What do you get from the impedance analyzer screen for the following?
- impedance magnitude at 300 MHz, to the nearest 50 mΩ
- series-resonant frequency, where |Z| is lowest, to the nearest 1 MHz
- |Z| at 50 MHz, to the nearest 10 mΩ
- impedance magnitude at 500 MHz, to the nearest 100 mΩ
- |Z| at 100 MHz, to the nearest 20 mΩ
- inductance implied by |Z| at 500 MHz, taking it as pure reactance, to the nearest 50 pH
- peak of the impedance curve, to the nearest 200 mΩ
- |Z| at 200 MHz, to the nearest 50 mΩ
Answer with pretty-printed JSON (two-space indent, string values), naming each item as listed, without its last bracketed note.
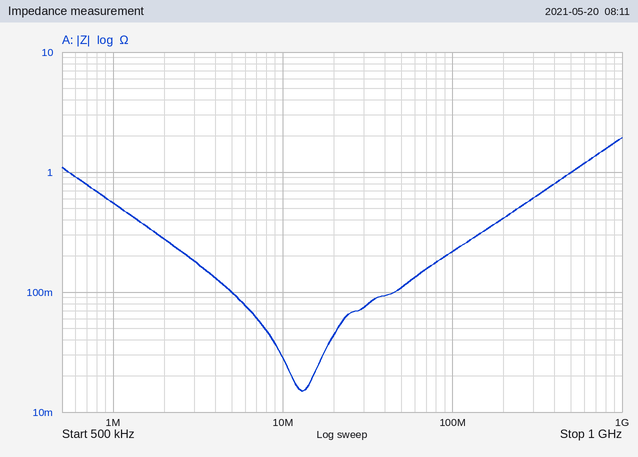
{
  "impedance magnitude at 300 MHz, to the nearest 50 mΩ": "600 mΩ",
  "series-resonant frequency, where |Z| is lowest, to the nearest 1 MHz": "13 MHz",
  "|Z| at 50 MHz, to the nearest 10 mΩ": "110 mΩ",
  "impedance magnitude at 500 MHz, to the nearest 100 mΩ": "1.0 Ω",
  "|Z| at 100 MHz, to the nearest 20 mΩ": "220 mΩ",
  "inductance implied by |Z| at 500 MHz, taking it as pure reactance, to the nearest 50 pH": "300 pH",
  "peak of the impedance curve, to the nearest 200 mΩ": "2.0 Ω",
  "|Z| at 200 MHz, to the nearest 50 mΩ": "400 mΩ"
}
